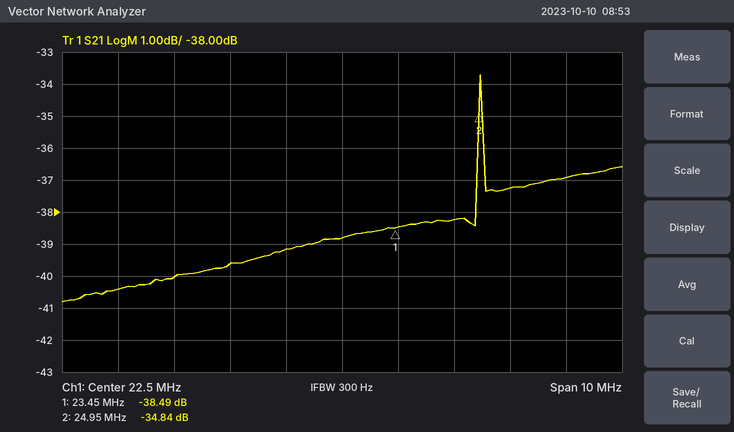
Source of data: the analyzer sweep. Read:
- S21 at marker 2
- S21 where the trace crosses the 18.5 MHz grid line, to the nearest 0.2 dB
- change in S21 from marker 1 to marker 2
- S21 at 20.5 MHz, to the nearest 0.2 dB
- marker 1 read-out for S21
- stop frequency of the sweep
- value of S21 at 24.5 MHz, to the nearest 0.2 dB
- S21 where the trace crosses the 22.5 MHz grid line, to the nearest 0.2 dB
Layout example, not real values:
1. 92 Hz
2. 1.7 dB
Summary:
1. -34.84 dB
2. -40.4 dB
3. 3.65 dB
4. -39.6 dB
5. -38.49 dB
6. 27.5 MHz
7. -38.2 dB
8. -38.8 dB
